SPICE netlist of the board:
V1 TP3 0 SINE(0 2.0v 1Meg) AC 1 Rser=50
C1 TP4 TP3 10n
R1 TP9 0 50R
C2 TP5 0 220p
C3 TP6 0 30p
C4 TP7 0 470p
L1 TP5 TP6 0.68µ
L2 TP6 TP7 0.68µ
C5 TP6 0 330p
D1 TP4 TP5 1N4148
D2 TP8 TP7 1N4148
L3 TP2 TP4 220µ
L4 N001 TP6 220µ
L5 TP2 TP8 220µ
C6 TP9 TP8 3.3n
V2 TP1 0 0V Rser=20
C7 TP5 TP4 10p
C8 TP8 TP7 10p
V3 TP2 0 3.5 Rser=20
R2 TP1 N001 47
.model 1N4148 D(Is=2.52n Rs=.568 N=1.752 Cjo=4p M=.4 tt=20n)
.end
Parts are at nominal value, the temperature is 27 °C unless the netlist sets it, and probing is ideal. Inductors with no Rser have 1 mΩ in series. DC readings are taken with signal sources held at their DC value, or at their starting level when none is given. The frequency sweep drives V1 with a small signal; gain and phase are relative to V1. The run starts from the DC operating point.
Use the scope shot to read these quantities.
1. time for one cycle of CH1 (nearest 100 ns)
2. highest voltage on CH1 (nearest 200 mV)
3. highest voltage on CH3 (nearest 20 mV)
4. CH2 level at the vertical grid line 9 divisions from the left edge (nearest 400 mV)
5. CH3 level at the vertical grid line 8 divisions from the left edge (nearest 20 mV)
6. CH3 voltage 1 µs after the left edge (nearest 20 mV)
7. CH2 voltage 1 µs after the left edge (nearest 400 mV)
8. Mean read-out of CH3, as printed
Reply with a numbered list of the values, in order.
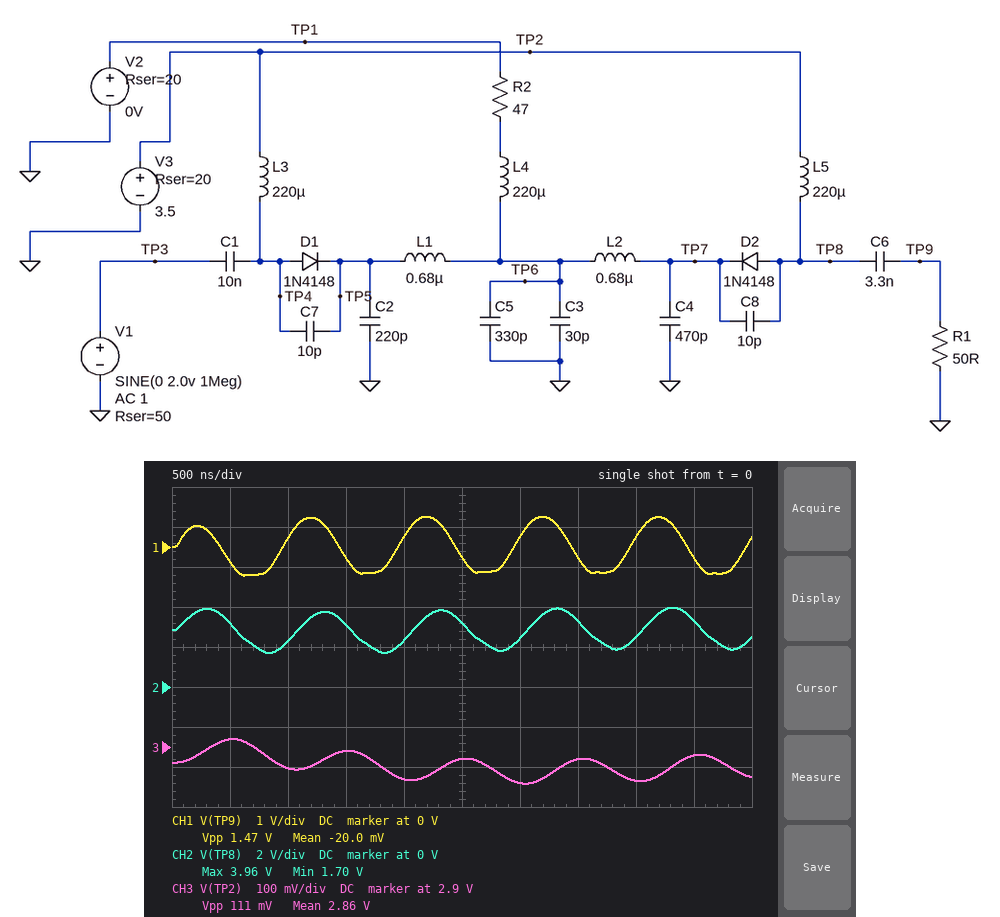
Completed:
1. 1.0 µs
2. 800 mV
3. 2.92 V
4. 3.2 V
5. 2.82 V
6. 2.84 V
7. 2.4 V
8. 2.86 V
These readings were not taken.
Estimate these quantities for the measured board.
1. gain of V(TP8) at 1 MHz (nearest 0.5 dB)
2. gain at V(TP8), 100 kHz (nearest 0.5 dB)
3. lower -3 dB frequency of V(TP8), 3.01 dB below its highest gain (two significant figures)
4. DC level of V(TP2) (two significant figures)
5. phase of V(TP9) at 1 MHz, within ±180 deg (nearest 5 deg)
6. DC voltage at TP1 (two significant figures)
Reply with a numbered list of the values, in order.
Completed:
1. -5.5 dB
2. -7.5 dB
3. 130 kHz
4. 2.9 V
5. 20 deg
6. 640 mV
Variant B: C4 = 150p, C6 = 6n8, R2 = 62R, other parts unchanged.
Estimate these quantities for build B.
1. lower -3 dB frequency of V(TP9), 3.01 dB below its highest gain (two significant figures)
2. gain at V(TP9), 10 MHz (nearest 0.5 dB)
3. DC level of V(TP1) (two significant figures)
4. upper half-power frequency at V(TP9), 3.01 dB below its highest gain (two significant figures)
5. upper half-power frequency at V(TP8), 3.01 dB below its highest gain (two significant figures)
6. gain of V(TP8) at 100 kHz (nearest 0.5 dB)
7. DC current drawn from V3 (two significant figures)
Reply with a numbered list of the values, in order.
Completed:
1. 300 kHz
2. -6.5 dB
3. 550 mV
4. 19 MHz
5. 280 kHz
6. -7.0 dB
7. 27 mA
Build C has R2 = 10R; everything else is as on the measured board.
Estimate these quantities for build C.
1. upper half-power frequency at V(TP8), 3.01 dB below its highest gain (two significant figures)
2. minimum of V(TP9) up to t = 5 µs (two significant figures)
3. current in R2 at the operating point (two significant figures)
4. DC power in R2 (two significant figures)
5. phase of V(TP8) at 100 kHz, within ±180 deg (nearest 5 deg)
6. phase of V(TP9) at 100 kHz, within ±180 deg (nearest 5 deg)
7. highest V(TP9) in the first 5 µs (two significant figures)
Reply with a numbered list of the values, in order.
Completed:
1. 270 kHz
2. -840 mV
3. 55 mA
4. 30 mW
5. 130 deg
6. -145 deg
7. 810 mV
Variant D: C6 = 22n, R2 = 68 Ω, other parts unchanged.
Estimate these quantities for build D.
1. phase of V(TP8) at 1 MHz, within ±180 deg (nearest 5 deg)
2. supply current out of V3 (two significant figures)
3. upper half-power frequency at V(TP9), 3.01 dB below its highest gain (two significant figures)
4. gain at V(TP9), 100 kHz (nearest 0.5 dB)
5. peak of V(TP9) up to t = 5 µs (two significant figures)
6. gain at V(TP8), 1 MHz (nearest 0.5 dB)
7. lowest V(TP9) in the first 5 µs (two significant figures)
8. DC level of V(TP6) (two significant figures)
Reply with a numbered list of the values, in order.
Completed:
1. -5 deg
2. 26 mA
3. 18 MHz
4. -13.5 dB
5. 690 mV
6. -7.0 dB
7. -690 mV
8. 2.3 V
